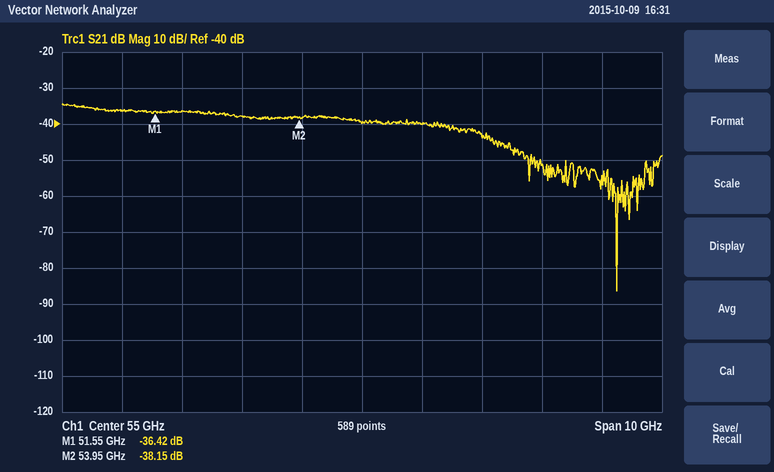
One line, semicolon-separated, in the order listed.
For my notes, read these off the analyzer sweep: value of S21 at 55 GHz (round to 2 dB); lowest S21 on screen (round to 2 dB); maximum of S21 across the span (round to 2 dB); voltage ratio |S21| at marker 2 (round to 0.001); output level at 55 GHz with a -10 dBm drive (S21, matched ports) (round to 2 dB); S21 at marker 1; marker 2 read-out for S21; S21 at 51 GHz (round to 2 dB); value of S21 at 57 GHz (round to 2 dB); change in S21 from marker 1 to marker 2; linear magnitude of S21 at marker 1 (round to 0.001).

-40 dB; -86 dB; -34 dB; 0.012; -50 dBm; -36.42 dB; -38.15 dB; -36 dB; -44 dB; -1.73 dB; 0.015
